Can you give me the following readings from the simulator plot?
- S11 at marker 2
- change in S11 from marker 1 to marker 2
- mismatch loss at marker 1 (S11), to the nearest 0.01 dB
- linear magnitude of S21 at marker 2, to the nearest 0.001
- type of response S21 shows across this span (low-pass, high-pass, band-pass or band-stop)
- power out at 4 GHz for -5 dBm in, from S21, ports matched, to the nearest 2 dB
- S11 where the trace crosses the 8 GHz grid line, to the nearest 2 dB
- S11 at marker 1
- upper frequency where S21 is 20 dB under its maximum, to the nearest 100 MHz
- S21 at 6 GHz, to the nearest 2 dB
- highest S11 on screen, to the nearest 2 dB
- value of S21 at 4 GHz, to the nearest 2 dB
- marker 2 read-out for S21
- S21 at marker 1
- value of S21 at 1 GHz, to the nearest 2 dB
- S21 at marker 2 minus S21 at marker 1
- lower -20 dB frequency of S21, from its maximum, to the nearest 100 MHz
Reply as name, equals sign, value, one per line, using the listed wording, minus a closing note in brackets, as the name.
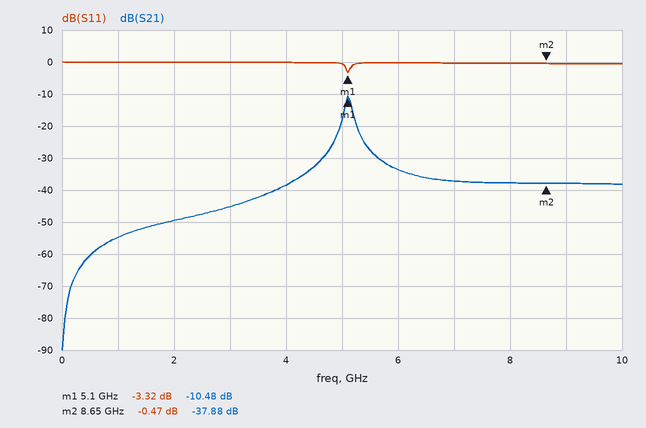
S11 at marker 2 = -0.47 dB
change in S11 from marker 1 to marker 2 = 2.85 dB
mismatch loss at marker 1 (S11), to the nearest 0.01 dB = 2.72 dB
linear magnitude of S21 at marker 2, to the nearest 0.001 = 0.013
type of response S21 shows across this span = band-pass
power out at 4 GHz for -5 dBm in, from S21, ports matched, to the nearest 2 dB = -44 dBm
S11 where the trace crosses the 8 GHz grid line, to the nearest 2 dB = 0 dB
S11 at marker 1 = -3.32 dB
upper frequency where S21 is 20 dB under its maximum, to the nearest 100 MHz = 5.7 GHz
S21 at 6 GHz, to the nearest 2 dB = -34 dB
highest S11 on screen, to the nearest 2 dB = 0 dB
value of S21 at 4 GHz, to the nearest 2 dB = -38 dB
marker 2 read-out for S21 = -37.88 dB
S21 at marker 1 = -10.48 dB
value of S21 at 1 GHz, to the nearest 2 dB = -54 dB
S21 at marker 2 minus S21 at marker 1 = -27.40 dB
lower -20 dB frequency of S21, from its maximum, to the nearest 100 MHz = 4.6 GHz
